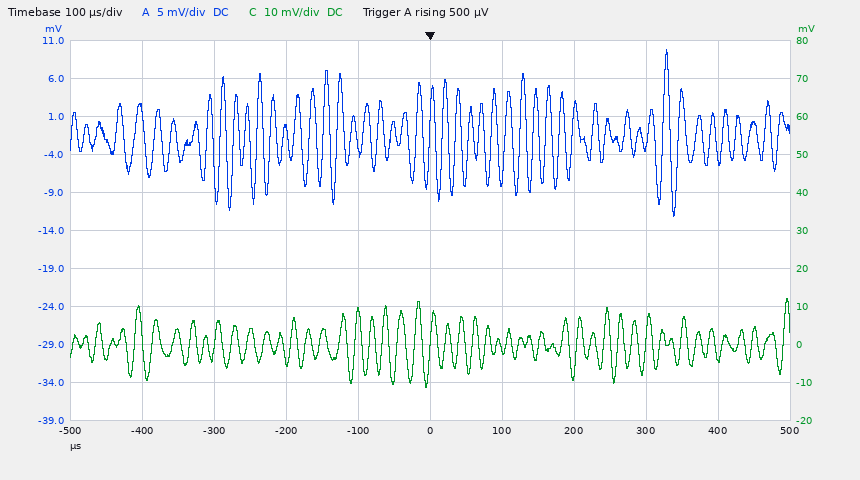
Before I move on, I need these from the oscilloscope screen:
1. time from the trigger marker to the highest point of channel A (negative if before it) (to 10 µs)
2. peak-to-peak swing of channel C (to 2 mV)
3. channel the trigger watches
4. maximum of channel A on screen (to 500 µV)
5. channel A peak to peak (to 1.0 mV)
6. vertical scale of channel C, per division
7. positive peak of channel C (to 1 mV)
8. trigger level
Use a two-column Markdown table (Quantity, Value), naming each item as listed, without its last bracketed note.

| Quantity | Value |
|---|---|
| time from the trigger marker to the highest point of channel A (negative if before it) | +330 µs |
| peak-to-peak swing of channel C | 24 mV |
| channel the trigger watches | channel A |
| maximum of channel A on screen | 10.0 mV |
| channel A peak to peak | 22.0 mV |
| vertical scale of channel C, per division | 10 mV |
| positive peak of channel C | 12 mV |
| trigger level | 500 µV |
